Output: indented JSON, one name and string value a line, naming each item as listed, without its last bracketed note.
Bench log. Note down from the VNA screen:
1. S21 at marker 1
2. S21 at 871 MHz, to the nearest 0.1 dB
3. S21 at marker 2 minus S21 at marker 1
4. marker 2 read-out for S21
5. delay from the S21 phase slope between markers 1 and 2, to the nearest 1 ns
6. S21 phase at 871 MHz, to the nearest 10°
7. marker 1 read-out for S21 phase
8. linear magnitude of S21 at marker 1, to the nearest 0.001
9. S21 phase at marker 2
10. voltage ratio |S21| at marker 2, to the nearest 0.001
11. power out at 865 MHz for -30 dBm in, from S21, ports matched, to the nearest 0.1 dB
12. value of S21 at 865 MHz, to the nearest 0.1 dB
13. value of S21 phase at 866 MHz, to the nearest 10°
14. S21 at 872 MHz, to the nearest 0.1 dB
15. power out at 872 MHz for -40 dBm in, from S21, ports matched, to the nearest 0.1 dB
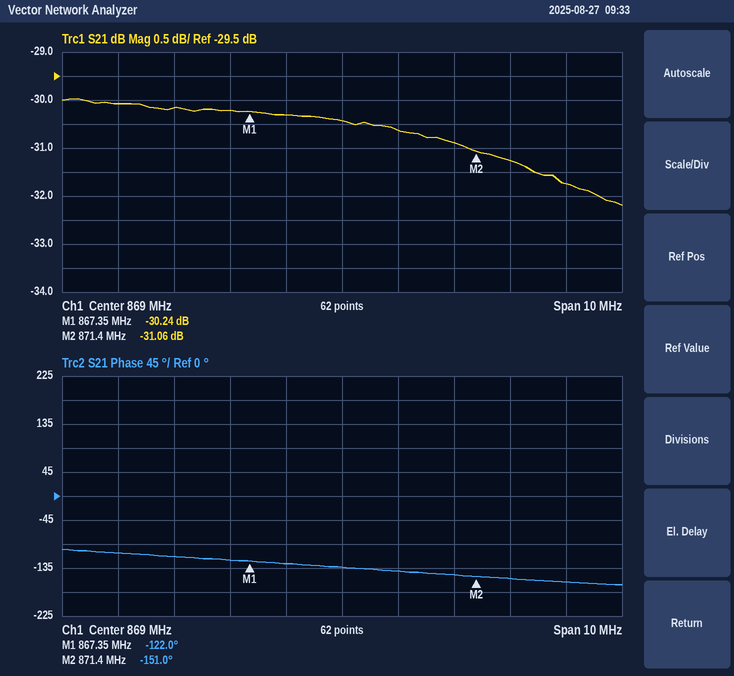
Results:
{
  "S21 at marker 1": "-30.24 dB",
  "S21 at 871 MHz, to the nearest 0.1 dB": "-30.9 dB",
  "S21 at marker 2 minus S21 at marker 1": "-0.82 dB",
  "marker 2 read-out for S21": "-31.06 dB",
  "delay from the S21 phase slope between markers 1 and 2, to the nearest 1 ns": "20 ns",
  "S21 phase at 871 MHz, to the nearest 10°": "-150°",
  "marker 1 read-out for S21 phase": "-122.0°",
  "linear magnitude of S21 at marker 1, to the nearest 0.001": "0.031",
  "S21 phase at marker 2": "-151.0°",
  "voltage ratio |S21| at marker 2, to the nearest 0.001": "0.028",
  "power out at 865 MHz for -30 dBm in, from S21, ports matched, to the nearest 0.1 dB": "-60.1 dBm",
  "value of S21 at 865 MHz, to the nearest 0.1 dB": "-30.1 dB",
  "value of S21 phase at 866 MHz, to the nearest 10°": "-110°",
  "S21 at 872 MHz, to the nearest 0.1 dB": "-31.3 dB",
  "power out at 872 MHz for -40 dBm in, from S21, ports matched, to the nearest 0.1 dB": "-71.3 dBm"
}
